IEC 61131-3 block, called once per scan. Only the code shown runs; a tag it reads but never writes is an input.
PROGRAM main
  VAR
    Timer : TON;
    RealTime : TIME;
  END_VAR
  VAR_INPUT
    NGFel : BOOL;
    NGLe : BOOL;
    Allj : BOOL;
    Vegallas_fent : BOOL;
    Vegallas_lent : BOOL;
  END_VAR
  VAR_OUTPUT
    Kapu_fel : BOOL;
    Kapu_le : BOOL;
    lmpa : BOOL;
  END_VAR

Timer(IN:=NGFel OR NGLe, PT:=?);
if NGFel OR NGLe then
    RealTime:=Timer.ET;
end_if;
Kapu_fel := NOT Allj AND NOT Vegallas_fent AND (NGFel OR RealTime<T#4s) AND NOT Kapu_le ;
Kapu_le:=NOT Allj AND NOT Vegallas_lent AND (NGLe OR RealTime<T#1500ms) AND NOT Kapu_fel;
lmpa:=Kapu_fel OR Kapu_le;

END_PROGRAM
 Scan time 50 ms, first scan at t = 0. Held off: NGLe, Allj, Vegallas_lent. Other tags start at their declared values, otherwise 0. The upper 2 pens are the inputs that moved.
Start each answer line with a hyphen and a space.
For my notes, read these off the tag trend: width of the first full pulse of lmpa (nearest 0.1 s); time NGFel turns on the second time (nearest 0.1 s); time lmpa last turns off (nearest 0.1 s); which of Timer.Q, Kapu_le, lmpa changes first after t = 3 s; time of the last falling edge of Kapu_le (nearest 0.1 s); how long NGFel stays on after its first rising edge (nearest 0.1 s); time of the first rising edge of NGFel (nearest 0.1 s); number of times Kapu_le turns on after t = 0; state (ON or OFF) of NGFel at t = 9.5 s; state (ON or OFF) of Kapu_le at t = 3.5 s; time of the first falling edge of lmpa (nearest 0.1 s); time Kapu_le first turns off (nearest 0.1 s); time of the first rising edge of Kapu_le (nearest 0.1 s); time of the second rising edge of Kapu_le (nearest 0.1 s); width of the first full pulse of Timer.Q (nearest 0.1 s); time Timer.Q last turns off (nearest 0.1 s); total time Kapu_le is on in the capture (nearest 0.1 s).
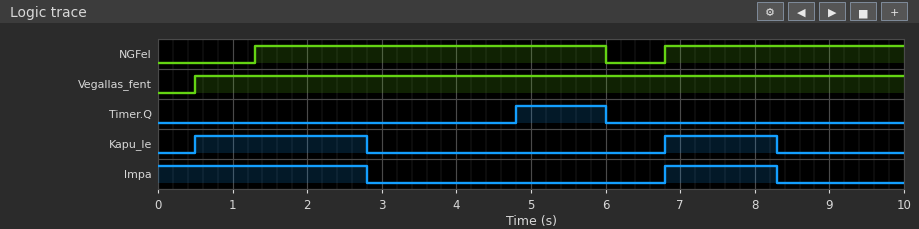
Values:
- 1.5 s
- 6.8 s
- 8.3 s
- Timer.Q
- 8.3 s
- 4.7 s
- 1.3 s
- 2
- ON
- OFF
- 2.8 s
- 2.8 s
- 0.5 s
- 6.8 s
- 1.2 s
- 6.0 s
- 3.8 s
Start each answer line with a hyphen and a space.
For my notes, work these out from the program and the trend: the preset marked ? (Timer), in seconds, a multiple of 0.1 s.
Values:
- 3.5 s
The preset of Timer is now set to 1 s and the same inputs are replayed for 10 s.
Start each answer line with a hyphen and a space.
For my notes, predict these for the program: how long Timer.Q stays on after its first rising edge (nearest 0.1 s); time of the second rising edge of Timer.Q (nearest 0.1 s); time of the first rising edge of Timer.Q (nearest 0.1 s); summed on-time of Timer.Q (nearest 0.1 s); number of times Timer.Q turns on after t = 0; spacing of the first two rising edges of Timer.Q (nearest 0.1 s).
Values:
- 3.7 s
- 7.8 s
- 2.3 s
- 5.9 s
- 2
- 5.5 s
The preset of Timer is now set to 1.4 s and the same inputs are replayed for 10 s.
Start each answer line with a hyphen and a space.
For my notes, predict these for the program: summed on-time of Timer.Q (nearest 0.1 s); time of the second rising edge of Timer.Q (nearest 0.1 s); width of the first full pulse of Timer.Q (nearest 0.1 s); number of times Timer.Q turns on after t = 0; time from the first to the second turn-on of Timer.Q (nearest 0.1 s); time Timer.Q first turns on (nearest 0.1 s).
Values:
- 5.1 s
- 8.2 s
- 3.3 s
- 2
- 5.5 s
- 2.7 s
